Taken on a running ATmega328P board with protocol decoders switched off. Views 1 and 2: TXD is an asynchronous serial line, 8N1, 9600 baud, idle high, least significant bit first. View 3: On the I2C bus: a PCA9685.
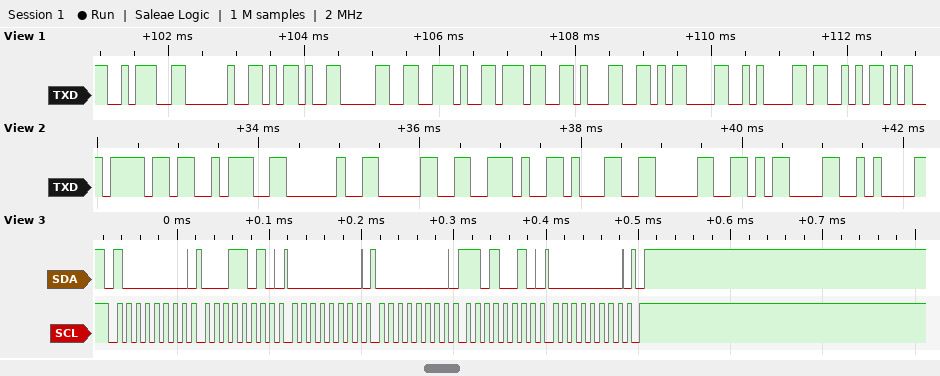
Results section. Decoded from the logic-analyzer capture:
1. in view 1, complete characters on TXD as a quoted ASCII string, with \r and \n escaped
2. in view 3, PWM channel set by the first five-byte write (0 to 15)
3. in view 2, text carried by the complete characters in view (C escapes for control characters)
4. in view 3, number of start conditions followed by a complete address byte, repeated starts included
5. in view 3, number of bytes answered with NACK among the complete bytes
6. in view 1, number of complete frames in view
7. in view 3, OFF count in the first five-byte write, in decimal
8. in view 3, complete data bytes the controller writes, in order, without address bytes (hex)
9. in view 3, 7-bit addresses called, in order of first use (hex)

": -0.71\r\nS"
5
"o: 0.10\r\n"
1
0
10
210
1A 00 00 D2 00
0x40
